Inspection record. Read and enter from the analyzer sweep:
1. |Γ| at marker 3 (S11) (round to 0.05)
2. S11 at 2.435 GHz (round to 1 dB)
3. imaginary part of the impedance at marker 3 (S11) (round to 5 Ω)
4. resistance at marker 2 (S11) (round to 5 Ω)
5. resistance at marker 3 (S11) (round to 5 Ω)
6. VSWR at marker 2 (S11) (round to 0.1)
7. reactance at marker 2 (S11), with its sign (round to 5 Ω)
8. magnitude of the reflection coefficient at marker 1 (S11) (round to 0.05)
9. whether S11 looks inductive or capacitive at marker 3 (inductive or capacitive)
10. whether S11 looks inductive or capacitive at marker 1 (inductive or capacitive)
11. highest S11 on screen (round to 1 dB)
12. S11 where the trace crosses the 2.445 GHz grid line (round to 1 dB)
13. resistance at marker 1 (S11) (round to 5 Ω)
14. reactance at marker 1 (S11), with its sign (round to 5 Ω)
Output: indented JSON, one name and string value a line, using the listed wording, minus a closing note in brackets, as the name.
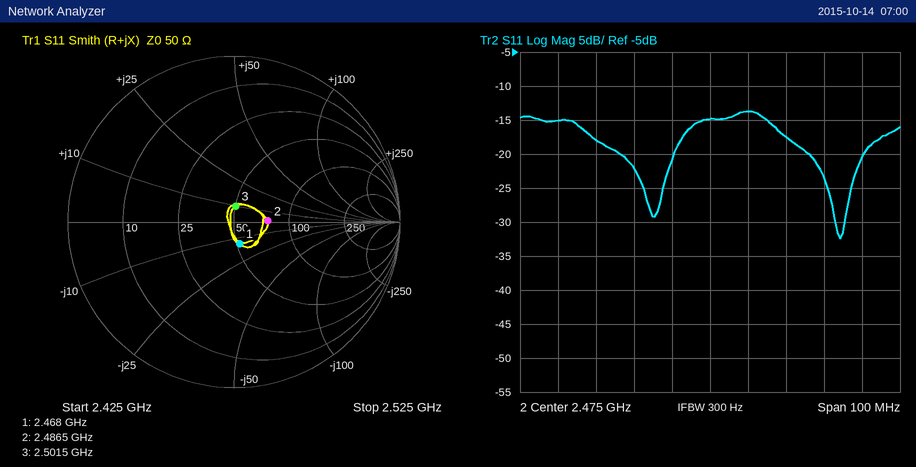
{
  "|Γ| at marker 3 (S11)": "0.10",
  "S11 at 2.435 GHz": "-15 dB",
  "imaginary part of the impedance at marker 3 (S11)": "+10 Ω",
  "resistance at marker 2 (S11)": "75 Ω",
  "resistance at marker 3 (S11)": "50 Ω",
  "VSWR at marker 2 (S11)": "1.5",
  "reactance at marker 2 (S11), with its sign": "0 Ω",
  "magnitude of the reflection coefficient at marker 1 (S11)": "0.15",
  "whether S11 looks inductive or capacitive at marker 3": "inductive",
  "whether S11 looks inductive or capacitive at marker 1": "capacitive",
  "highest S11 on screen": "-14 dB",
  "S11 where the trace crosses the 2.445 GHz grid line": "-18 dB",
  "resistance at marker 1 (S11)": "50 Ω",
  "reactance at marker 1 (S11), with its sign": "-15 Ω"
}
